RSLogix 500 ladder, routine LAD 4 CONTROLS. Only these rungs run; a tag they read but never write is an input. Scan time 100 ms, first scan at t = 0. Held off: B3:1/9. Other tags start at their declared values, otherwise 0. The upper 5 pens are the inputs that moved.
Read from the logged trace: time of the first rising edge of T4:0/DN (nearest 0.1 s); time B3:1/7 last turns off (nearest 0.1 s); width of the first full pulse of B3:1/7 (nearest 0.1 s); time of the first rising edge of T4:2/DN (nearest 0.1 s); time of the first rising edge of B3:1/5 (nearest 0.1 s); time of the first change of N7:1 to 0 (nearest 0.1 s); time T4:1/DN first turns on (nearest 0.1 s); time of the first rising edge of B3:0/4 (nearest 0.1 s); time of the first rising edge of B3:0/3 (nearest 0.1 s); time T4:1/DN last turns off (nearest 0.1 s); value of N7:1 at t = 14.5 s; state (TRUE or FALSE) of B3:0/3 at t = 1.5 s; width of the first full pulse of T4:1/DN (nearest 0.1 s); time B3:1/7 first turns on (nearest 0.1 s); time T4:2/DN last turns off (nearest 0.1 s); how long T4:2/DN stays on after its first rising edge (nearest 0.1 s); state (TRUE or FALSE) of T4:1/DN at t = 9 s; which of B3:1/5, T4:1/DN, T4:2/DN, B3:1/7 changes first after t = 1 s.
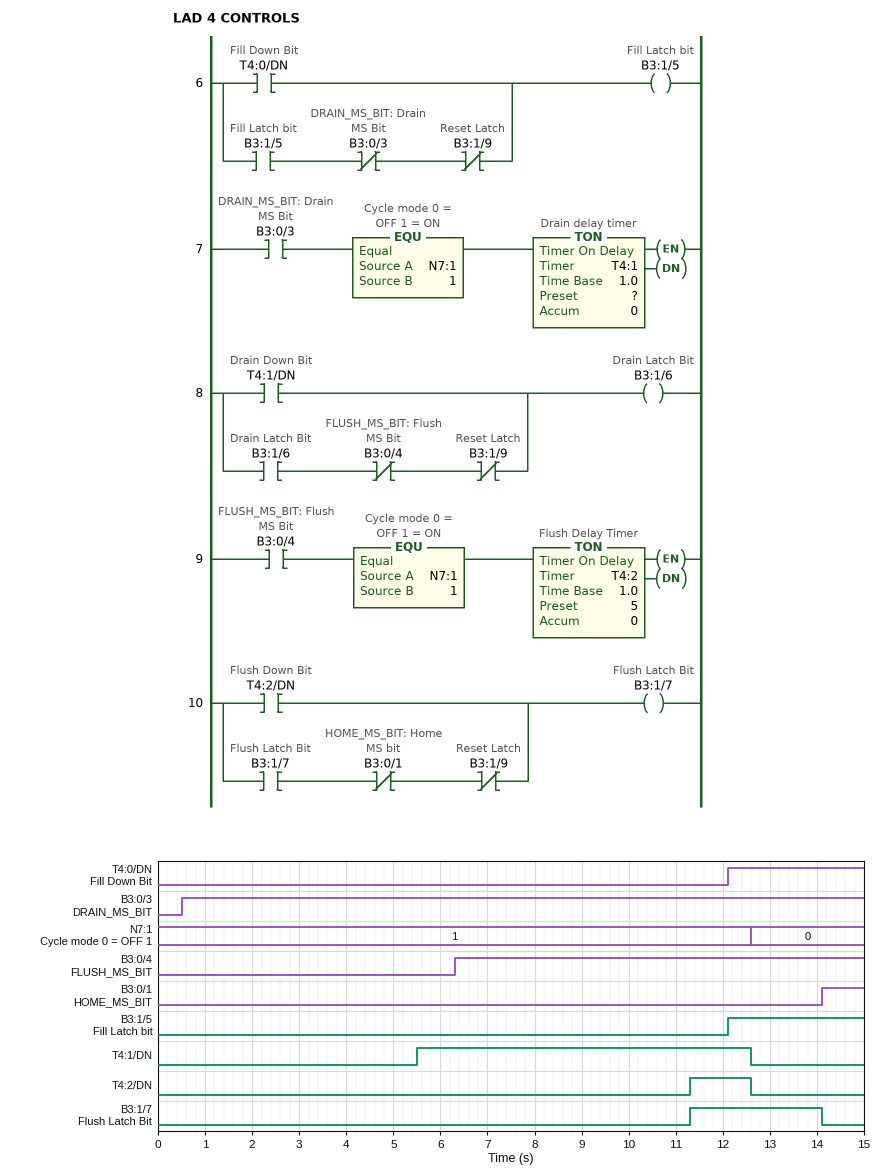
12.1 s
14.1 s
2.8 s
11.3 s
12.1 s
12.6 s
5.5 s
6.3 s
0.5 s
12.6 s
0
TRUE
7.1 s
11.3 s
12.6 s
1.3 s
TRUE
T4:1/DN
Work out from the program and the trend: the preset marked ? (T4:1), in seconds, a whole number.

5 s
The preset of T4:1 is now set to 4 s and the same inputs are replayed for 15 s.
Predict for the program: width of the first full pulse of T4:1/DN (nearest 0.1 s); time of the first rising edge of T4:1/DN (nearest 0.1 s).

8.1 s
4.5 s
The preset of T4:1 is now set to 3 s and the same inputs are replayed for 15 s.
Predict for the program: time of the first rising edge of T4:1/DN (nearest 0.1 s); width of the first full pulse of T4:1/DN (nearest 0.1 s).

3.5 s
9.1 s
